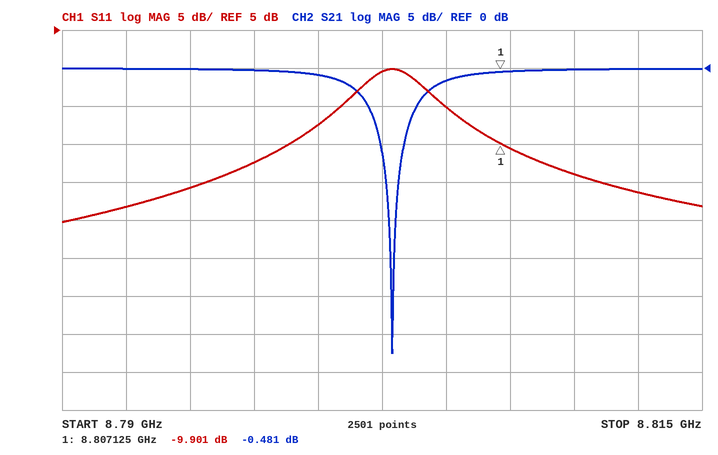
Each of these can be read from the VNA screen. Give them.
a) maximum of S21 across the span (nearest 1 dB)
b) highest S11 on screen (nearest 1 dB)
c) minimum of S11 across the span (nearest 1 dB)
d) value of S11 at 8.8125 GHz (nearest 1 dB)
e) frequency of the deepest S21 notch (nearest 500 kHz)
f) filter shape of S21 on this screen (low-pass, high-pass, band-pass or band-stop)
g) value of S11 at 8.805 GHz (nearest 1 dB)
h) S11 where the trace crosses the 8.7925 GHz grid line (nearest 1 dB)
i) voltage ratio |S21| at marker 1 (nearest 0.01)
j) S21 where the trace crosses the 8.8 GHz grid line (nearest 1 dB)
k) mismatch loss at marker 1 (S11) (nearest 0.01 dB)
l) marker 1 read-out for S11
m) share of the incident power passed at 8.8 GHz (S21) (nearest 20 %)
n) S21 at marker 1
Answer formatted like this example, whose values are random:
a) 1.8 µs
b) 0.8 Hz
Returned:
a) 0 dB
b) 0 dB
c) -20 dB
d) -16 dB
e) 8.8030 GHz
f) band-stop
g) -5 dB
h) -18 dB
i) 0.95
j) -1 dB
k) 0.47 dB
l) -9.901 dB
m) 80 %
n) -0.481 dB
